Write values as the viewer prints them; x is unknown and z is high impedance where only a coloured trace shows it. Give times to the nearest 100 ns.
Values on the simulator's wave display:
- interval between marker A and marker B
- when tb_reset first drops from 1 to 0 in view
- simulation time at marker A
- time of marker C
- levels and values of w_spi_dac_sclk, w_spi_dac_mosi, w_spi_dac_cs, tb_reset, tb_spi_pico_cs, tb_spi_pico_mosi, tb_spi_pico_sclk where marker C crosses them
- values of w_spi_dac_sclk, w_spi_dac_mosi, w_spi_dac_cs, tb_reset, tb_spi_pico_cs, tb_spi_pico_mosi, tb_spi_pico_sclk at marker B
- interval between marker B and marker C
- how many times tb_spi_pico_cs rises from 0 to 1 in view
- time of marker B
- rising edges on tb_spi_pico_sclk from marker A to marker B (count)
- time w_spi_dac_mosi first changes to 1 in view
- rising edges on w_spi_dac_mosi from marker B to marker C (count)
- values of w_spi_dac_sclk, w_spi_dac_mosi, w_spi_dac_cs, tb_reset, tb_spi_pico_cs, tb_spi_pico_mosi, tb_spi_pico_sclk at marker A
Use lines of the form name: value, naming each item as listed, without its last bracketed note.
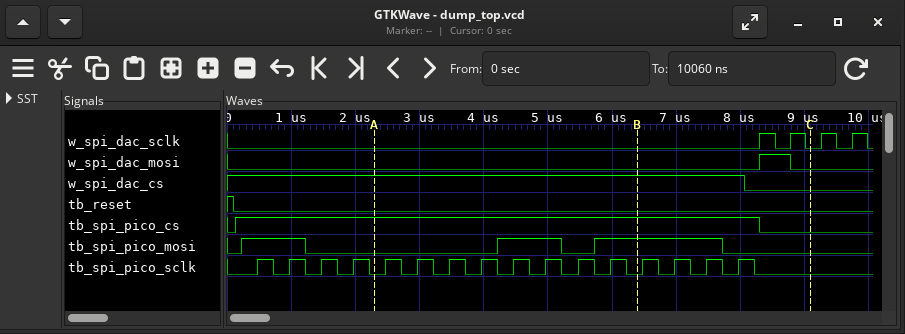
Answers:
interval between marker A and marker B: 4100 ns
when tb_reset first drops from 1 to 0 in view: 100 ns
simulation time at marker A: 2300 ns
time of marker C: 9100 ns
levels and values of w_spi_dac_sclk, w_spi_dac_mosi, w_spi_dac_cs, tb_reset, tb_spi_pico_cs, tb_spi_pico_mosi, tb_spi_pico_sclk where marker C crosses them: w_spi_dac_sclk=0, w_spi_dac_mosi=0, w_spi_dac_cs=0, tb_reset=0, tb_spi_pico_cs=0, tb_spi_pico_mosi=0, tb_spi_pico_sclk=0
values of w_spi_dac_sclk, w_spi_dac_mosi, w_spi_dac_cs, tb_reset, tb_spi_pico_cs, tb_spi_pico_mosi, tb_spi_pico_sclk at marker B: w_spi_dac_sclk=0, w_spi_dac_mosi=0, w_spi_dac_cs=1, tb_reset=0, tb_spi_pico_cs=1, tb_spi_pico_mosi=1, tb_spi_pico_sclk=0
interval between marker B and marker C: 2700 ns
how many times tb_spi_pico_cs rises from 0 to 1 in view: 1
time of marker B: 6400 ns
rising edges on tb_spi_pico_sclk from marker A to marker B: 8
time w_spi_dac_mosi first changes to 1 in view: 8300 ns
rising edges on w_spi_dac_mosi from marker B to marker C: 1
values of w_spi_dac_sclk, w_spi_dac_mosi, w_spi_dac_cs, tb_reset, tb_spi_pico_cs, tb_spi_pico_mosi, tb_spi_pico_sclk at marker A: w_spi_dac_sclk=0, w_spi_dac_mosi=0, w_spi_dac_cs=1, tb_reset=0, tb_spi_pico_cs=1, tb_spi_pico_mosi=0, tb_spi_pico_sclk=0
